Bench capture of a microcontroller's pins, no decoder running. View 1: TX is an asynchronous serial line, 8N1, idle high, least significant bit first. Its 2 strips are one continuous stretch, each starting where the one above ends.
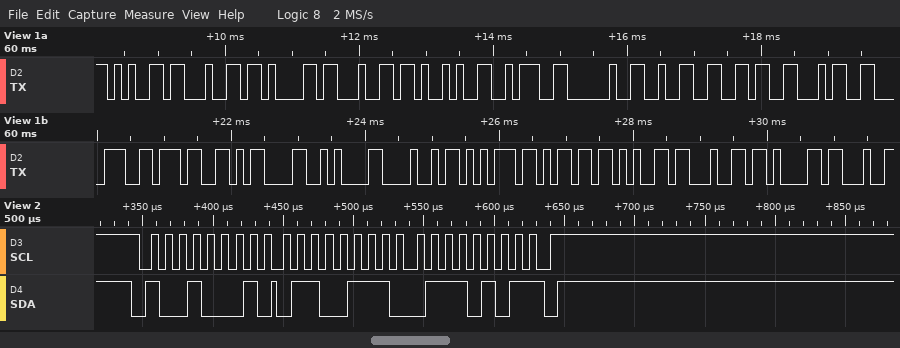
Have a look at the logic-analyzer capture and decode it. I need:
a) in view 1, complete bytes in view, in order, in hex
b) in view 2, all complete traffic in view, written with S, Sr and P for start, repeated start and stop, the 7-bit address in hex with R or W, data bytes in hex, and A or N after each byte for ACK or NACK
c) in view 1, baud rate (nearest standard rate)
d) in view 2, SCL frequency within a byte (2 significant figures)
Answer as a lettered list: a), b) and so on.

a) 65 64 61 64 29 3A 20 32 36 34 38 37 0D 0A 48 75 6D 65 64 61
b) S 48R A 67 A 75 N P
c) 9600 baud
d) 100 kHz
